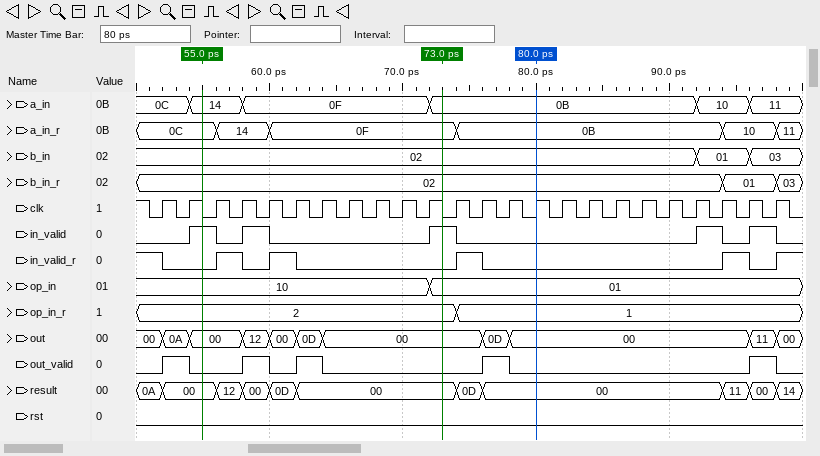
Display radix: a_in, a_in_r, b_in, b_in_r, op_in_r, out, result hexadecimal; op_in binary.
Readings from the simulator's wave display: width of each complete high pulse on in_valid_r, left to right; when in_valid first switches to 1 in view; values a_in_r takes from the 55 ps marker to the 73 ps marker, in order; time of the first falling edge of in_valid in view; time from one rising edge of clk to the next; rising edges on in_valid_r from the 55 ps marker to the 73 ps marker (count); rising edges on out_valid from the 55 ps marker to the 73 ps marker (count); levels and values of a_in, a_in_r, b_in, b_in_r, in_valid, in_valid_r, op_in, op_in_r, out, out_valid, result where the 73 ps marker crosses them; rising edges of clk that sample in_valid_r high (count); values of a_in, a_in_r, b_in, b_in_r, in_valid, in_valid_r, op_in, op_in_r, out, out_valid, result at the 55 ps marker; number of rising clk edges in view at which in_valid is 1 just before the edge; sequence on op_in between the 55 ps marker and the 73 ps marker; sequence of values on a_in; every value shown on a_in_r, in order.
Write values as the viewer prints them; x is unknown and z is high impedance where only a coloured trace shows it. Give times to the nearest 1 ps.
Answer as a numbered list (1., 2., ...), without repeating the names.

1. 2 ps, 2 ps, 2 ps, 2 ps
2. 54 ps
3. 0C, 14, 0F
4. 56 ps
5. 2 ps
6. 2
7. 2
8. a_in=0B, a_in_r=0F, b_in=02, b_in_r=02, in_valid=1, in_valid_r=0, op_in=01, op_in_r=2, out=00, out_valid=0, result=00
9. 5
10. a_in=14, a_in_r=0C, b_in=02, b_in_r=02, in_valid=1, in_valid_r=0, op_in=10, op_in_r=2, out=00, out_valid=0, result=00
11. 5
12. 10, 01
13. 0C, 14, 0F, 0B, 10, 11
14. 0C, 14, 0F, 0B, 10, 11
